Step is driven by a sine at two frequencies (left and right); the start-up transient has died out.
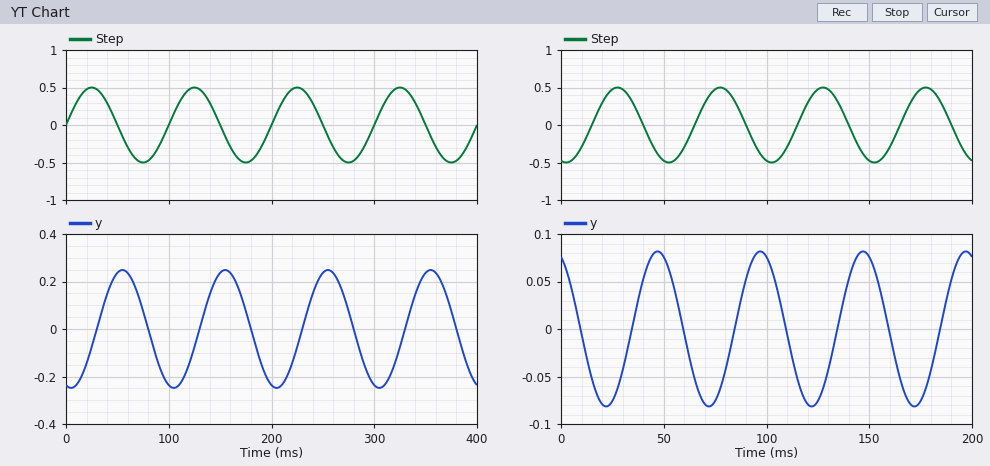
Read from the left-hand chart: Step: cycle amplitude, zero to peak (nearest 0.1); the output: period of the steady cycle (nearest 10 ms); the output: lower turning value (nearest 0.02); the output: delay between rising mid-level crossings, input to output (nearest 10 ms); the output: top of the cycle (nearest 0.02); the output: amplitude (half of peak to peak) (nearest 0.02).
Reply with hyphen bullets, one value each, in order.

- 0.5
- 100 ms
- -0.24
- 30 ms
- 0.24
- 0.24
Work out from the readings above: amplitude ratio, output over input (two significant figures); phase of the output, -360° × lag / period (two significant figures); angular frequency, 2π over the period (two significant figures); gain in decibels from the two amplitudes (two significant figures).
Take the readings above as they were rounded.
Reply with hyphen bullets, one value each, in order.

- 0.48
- -110°
- 0.063 rad/ms
- -6.4 dB
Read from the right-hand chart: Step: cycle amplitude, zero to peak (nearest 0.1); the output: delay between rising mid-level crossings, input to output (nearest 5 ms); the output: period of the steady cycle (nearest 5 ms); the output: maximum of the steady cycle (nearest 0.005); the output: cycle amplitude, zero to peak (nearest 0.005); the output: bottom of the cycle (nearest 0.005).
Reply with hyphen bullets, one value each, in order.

- 0.5
- 20 ms
- 50 ms
- 0.080
- 0.080
- -0.080
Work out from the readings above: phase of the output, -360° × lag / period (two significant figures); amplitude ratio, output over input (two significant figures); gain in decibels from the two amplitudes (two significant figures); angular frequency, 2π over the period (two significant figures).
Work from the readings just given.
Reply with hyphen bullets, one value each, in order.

- -140°
- 0.16
- -16 dB
- 0.13 rad/ms
